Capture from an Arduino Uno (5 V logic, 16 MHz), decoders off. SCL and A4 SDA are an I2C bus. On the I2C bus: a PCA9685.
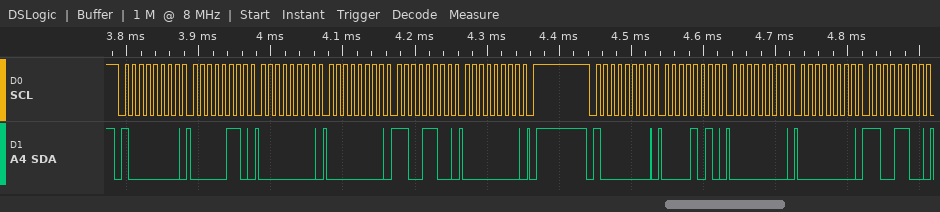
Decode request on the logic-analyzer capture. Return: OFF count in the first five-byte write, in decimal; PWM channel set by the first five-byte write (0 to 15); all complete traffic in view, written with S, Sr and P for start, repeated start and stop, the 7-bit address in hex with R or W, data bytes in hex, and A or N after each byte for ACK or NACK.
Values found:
204
0
S 40W A 06 A 00 A 00 A CC A 00 A P S 40W A 0A A 00 A 00 A CC A
